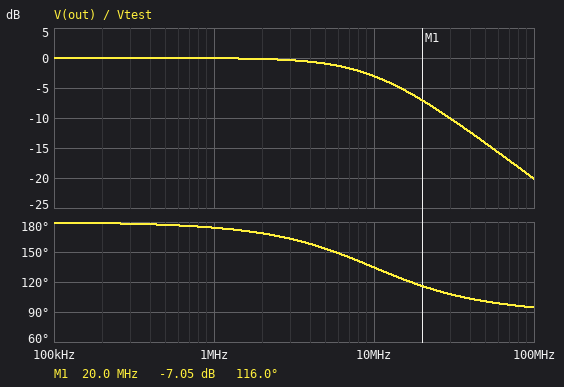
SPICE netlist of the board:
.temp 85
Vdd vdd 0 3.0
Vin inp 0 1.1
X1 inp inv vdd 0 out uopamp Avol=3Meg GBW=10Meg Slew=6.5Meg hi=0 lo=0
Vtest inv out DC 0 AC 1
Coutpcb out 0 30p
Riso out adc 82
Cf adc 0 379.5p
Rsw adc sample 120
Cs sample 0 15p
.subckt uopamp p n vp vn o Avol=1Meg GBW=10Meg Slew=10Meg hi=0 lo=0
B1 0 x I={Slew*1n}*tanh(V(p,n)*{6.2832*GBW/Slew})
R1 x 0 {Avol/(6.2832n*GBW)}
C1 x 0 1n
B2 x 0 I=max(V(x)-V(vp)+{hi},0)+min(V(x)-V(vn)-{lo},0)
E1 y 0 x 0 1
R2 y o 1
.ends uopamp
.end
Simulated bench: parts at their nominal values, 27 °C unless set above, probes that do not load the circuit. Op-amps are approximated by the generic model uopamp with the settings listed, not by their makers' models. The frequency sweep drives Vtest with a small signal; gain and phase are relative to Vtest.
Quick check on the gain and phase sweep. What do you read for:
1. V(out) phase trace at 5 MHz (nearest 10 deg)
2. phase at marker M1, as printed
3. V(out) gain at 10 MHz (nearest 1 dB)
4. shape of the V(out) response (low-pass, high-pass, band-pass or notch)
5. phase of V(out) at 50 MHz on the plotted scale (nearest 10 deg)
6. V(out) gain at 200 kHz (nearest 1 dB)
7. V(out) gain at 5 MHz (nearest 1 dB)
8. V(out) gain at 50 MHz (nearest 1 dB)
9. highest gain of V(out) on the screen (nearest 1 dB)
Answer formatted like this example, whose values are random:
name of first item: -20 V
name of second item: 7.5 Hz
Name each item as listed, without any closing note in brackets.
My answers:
V(out) phase trace at 5 MHz: 150 deg
phase at marker M1, as printed: 116.0 deg
V(out) gain at 10 MHz: -3 dB
shape of the V(out) response: low-pass
phase of V(out) at 50 MHz on the plotted scale: 100 deg
V(out) gain at 200 kHz: 0 dB
V(out) gain at 5 MHz: -1 dB
V(out) gain at 50 MHz: -14 dB
highest gain of V(out) on the screen: 0 dB
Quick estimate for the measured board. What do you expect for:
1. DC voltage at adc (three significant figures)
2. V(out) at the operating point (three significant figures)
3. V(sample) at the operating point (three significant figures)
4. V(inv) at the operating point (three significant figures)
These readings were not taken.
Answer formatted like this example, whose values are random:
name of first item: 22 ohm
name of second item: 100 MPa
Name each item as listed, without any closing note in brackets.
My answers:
DC voltage at adc: 1.10 V
V(out) at the operating point: 1.10 V
V(sample) at the operating point: 1.10 V
V(inv) at the operating point: 1.10 V
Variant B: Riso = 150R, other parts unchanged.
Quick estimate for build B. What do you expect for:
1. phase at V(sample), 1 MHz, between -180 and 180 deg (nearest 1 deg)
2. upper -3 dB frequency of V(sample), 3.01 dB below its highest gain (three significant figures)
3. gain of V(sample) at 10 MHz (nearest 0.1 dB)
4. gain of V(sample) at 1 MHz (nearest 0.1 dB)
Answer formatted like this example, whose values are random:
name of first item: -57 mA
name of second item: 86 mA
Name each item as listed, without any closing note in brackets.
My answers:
phase at V(sample), 1 MHz, between -180 and 180 deg: 153 deg
upper -3 dB frequency of V(sample), 3.01 dB below its highest gain: 2.52 MHz
gain of V(sample) at 10 MHz: -14.8 dB
gain of V(sample) at 1 MHz: -0.6 dB
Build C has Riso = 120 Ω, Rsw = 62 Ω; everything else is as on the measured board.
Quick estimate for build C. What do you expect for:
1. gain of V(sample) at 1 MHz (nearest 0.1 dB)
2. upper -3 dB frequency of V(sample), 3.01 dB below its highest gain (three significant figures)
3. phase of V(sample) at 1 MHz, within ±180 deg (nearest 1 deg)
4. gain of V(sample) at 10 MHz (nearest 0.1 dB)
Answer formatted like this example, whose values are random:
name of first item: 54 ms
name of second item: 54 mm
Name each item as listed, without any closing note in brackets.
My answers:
gain of V(sample) at 1 MHz: -0.4 dB
upper -3 dB frequency of V(sample), 3.01 dB below its highest gain: 3.06 MHz
phase of V(sample) at 1 MHz, within ±180 deg: 157 deg
gain of V(sample) at 10 MHz: -13.0 dB
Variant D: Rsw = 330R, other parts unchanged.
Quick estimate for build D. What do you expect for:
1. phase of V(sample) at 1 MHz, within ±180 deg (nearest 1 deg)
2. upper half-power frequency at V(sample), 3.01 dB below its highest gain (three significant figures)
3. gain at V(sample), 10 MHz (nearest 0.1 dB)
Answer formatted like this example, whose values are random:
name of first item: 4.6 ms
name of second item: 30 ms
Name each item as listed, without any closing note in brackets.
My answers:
phase of V(sample) at 1 MHz, within ±180 deg: 161 deg
upper half-power frequency at V(sample), 3.01 dB below its highest gain: 4.08 MHz
gain at V(sample), 10 MHz: -10.5 dB
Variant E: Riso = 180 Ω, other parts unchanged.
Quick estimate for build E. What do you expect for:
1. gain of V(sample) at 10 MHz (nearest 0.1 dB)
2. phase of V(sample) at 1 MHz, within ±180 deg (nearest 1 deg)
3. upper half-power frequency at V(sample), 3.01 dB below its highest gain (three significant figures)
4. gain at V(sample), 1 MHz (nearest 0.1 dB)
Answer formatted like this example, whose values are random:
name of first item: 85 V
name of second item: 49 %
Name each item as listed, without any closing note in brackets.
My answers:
gain of V(sample) at 10 MHz: -16.3 dB
phase of V(sample) at 1 MHz, within ±180 deg: 150 deg
upper half-power frequency at V(sample), 3.01 dB below its highest gain: 2.14 MHz
gain at V(sample), 1 MHz: -0.8 dB
